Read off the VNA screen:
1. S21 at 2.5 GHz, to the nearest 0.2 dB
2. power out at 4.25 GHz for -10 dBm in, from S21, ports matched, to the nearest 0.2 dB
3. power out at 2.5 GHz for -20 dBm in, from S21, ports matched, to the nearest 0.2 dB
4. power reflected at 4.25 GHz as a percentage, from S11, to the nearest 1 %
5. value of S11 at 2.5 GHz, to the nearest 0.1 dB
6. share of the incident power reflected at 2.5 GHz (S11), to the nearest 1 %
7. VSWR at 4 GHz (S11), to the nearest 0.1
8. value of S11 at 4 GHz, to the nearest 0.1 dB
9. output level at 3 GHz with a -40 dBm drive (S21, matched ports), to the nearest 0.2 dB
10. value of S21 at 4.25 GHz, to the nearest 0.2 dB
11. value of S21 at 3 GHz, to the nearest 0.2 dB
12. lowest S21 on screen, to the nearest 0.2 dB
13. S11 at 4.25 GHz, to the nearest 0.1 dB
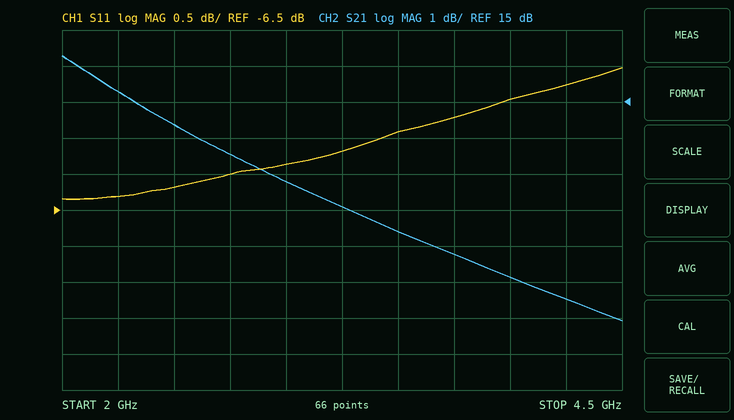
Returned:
14.4 dB
-0.4 dBm
-5.6 dBm
33 %
-6.2 dB
24 %
3.6
-5.0 dB
-27.2 dBm
9.6 dB
12.8 dB
9.0 dB
-4.8 dB
